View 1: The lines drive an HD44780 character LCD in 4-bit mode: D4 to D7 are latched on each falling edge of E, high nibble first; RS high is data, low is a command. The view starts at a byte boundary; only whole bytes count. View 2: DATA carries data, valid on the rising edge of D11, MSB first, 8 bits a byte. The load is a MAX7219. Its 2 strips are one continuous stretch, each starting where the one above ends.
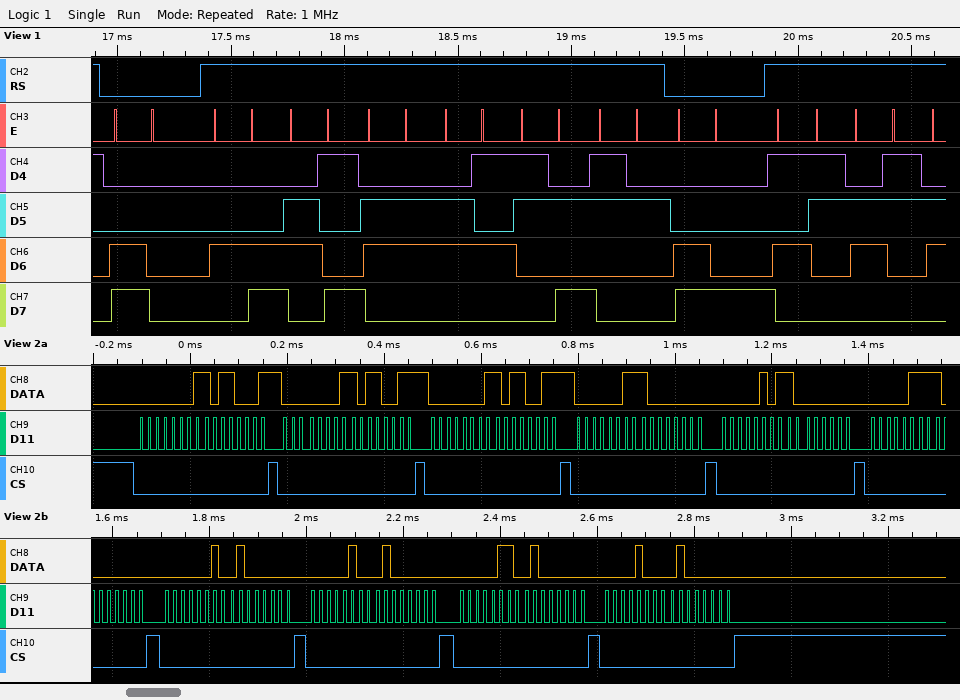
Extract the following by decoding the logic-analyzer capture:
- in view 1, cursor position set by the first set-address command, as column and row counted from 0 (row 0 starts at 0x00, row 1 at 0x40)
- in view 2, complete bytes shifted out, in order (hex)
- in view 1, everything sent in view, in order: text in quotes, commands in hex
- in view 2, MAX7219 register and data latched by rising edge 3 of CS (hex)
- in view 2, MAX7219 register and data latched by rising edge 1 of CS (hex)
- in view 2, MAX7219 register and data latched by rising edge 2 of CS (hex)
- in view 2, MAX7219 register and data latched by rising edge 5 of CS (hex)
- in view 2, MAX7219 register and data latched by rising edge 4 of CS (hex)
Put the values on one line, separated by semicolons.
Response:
column 0, row 1; 01 B1 01 B3 01 B3 03 80 05 80 07 80 02 40 04 40 06 40 08 40; 0xC0 "Life:2" 0xC8 "Sc"; register 0x1, data 0xB3; register 0x1, data 0xB1; register 0x1, data 0xB3; register 0x5, data 0x80; register 0x3, data 0x80
